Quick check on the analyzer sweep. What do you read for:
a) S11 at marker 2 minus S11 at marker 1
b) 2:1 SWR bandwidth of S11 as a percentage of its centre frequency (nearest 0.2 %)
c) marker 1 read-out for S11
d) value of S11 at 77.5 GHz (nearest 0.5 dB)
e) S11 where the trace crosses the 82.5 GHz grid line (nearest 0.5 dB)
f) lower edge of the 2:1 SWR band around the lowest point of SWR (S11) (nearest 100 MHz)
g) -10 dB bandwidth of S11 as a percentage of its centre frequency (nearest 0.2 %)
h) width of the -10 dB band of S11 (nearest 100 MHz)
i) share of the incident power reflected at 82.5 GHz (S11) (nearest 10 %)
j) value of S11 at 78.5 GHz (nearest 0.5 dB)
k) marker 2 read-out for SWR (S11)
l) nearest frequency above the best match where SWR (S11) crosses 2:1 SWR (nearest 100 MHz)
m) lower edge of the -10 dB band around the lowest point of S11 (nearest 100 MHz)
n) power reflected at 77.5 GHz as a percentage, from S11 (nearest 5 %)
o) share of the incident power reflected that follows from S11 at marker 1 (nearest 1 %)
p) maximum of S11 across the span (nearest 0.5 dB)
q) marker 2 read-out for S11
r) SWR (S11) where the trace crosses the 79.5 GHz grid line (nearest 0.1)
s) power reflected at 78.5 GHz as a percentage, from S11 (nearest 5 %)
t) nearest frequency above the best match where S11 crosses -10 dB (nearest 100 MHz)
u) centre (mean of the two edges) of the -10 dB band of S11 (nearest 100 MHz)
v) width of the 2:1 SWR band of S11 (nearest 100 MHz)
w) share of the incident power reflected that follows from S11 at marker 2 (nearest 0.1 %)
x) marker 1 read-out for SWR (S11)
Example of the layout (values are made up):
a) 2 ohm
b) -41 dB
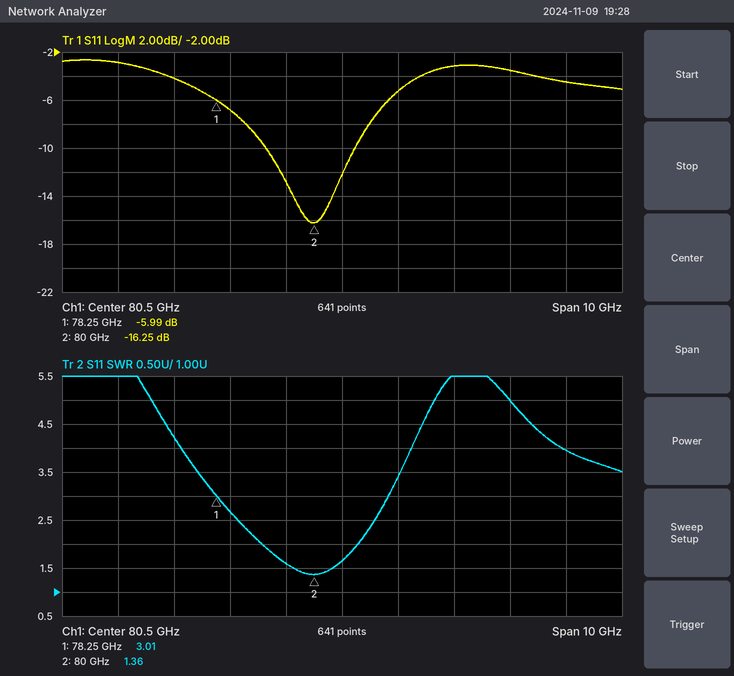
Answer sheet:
a) -10.26 dB
b) 2.2 %
c) -5.99 dB
d) -4.0 dB
e) -3.0 dB
f) 79.1 GHz
g) 2.0 %
h) 1.6 GHz
i) 50 %
j) -7.0 dB
k) 1.36
l) 80.8 GHz
m) 79.1 GHz
n) 40 %
o) 25 %
p) -2.5 dB
q) -16.25 dB
r) 1.6
s) 20 %
t) 80.7 GHz
u) 79.9 GHz
v) 1.7 GHz
w) 2.4 %
x) 3.01
